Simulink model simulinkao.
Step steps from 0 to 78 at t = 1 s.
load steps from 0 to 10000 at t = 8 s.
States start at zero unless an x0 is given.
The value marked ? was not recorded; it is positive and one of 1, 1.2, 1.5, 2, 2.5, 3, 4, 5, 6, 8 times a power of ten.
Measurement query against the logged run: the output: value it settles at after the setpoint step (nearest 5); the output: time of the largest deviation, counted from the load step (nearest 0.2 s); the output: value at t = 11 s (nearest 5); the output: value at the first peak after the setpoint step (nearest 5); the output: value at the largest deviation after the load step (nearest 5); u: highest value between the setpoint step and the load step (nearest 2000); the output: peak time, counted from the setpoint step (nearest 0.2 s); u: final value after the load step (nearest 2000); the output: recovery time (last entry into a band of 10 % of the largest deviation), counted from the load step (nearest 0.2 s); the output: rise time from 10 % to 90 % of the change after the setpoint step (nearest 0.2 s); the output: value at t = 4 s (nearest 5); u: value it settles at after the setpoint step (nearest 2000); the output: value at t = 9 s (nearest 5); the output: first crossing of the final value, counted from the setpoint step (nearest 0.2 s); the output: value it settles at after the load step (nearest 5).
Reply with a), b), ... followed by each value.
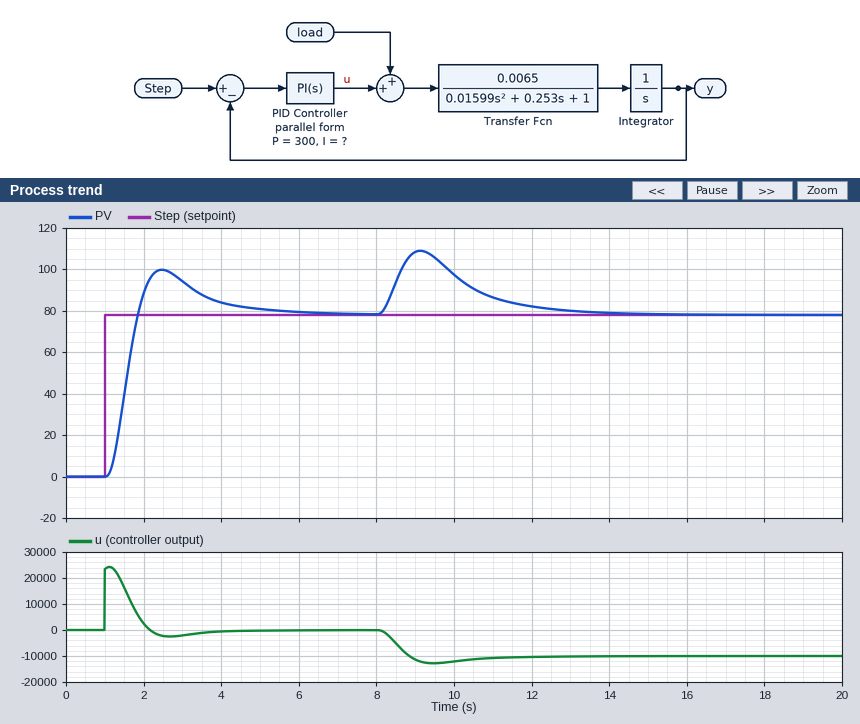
a) 80
b) 1.2 s
c) 85
d) 100
e) 110
f) 24000
g) 1.4 s
h) -10000
i) 4.4 s
j) 0.6 s
k) 85
l) 0
m) 110
n) 0.8 s
o) 80
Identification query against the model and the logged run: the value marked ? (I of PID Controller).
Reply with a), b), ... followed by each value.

a) 150
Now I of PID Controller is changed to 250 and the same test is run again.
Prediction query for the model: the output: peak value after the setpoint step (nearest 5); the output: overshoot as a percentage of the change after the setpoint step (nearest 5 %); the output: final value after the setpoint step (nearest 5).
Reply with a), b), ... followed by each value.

a) 110
b) 40 %
c) 80
